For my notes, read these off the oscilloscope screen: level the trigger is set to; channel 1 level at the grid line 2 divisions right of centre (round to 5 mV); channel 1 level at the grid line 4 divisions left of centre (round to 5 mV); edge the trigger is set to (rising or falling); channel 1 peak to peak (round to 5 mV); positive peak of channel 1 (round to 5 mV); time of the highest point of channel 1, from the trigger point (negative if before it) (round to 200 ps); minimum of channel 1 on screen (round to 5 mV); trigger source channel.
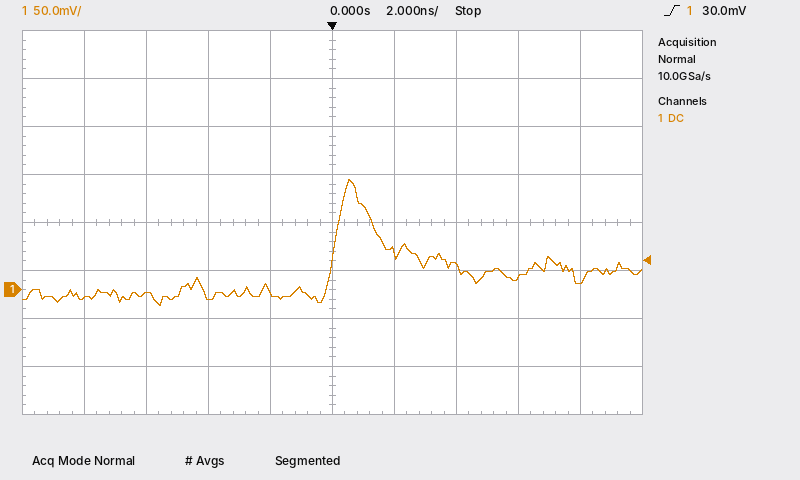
30.0 mV
25 mV
-10 mV
rising
130 mV
115 mV
+600 ps
-15 mV
channel 1
